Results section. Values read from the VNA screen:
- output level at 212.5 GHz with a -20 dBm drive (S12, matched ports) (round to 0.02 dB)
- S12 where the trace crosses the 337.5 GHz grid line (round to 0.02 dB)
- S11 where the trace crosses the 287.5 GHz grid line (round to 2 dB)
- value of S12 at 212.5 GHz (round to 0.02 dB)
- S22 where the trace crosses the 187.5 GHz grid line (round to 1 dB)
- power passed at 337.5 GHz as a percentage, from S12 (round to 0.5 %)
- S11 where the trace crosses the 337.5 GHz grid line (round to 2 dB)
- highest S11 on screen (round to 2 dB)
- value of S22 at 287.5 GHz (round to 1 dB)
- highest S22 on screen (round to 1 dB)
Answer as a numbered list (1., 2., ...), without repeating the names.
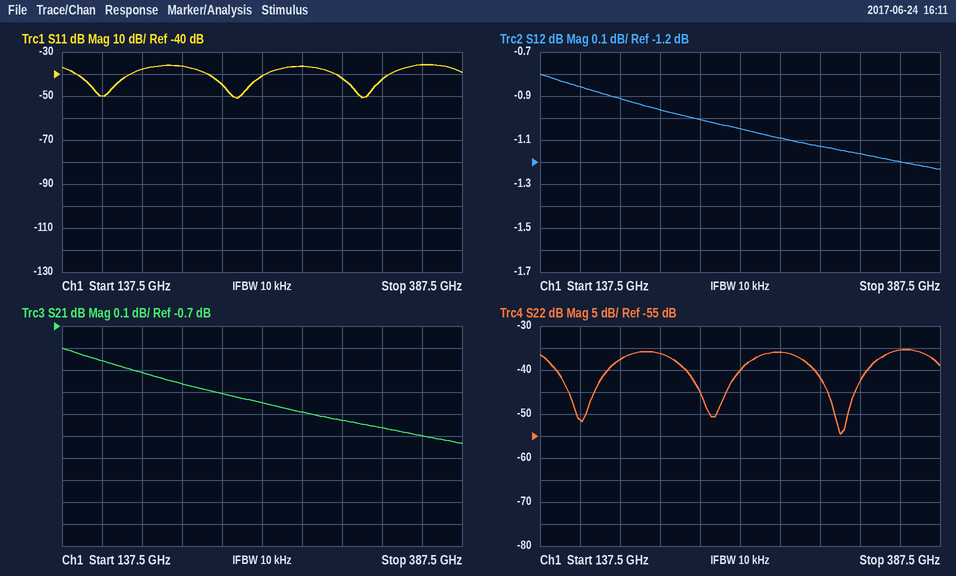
1. -20.96 dBm
2. -1.16 dB
3. -36 dB
4. -0.96 dB
5. -38 dB
6. 76.5 %
7. -42 dB
8. -36 dB
9. -36 dB
10. -35 dB
